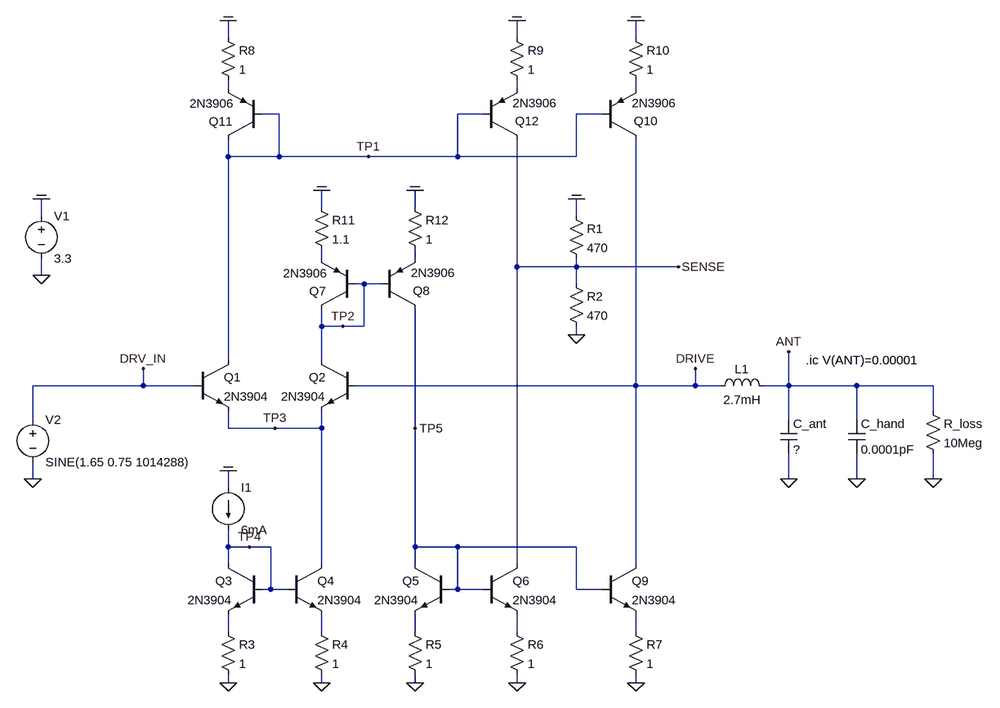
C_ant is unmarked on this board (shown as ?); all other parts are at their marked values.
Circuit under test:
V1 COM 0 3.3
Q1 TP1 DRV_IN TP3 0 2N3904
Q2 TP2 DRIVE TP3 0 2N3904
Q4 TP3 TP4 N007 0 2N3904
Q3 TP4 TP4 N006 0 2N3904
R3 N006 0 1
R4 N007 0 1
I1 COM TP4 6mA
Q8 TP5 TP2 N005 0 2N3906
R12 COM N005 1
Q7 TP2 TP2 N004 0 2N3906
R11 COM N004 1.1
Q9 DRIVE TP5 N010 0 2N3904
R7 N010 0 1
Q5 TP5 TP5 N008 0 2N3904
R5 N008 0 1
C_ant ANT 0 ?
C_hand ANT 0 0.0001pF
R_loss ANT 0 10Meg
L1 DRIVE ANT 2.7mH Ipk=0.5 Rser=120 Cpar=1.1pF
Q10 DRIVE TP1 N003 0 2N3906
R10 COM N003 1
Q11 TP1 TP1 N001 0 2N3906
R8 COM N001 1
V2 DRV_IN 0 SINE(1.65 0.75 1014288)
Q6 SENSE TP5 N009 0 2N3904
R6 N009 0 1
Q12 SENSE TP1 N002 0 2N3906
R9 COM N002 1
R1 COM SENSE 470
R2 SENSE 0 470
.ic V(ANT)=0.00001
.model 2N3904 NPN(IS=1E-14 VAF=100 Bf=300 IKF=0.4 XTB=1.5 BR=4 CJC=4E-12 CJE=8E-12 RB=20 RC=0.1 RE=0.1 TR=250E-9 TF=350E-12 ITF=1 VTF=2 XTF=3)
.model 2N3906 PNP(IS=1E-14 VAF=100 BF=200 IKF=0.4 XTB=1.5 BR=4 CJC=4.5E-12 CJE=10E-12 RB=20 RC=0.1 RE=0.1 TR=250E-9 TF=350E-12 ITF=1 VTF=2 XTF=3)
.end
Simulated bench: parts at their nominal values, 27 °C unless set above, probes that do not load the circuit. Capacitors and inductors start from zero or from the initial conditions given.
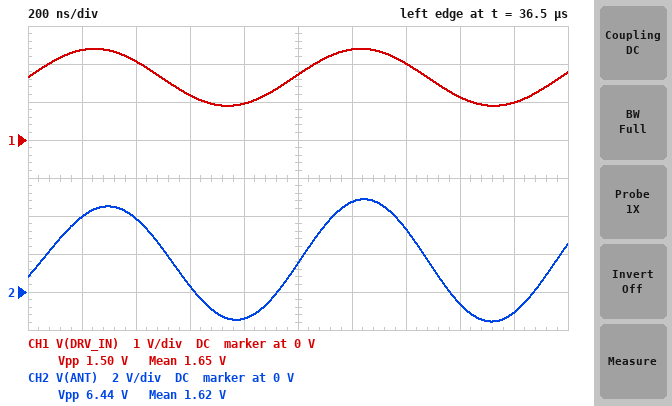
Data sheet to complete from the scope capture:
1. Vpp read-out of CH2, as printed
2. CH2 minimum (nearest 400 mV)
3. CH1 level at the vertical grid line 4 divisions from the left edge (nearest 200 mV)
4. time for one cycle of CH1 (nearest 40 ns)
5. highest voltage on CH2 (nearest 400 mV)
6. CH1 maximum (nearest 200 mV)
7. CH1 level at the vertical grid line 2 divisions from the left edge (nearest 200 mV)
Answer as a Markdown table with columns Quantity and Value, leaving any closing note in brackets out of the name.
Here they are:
| Quantity | Value |
|---|---|
| Vpp read-out of CH2, as printed | 6.44 V |
| CH2 minimum | -1.6 V |
| CH1 level at the vertical grid line 4 divisions from the left edge | 1.0 V |
| time for one cycle of CH1 | 1.00 µs |
| highest voltage on CH2 | 4.8 V |
| CH1 maximum | 2.4 V |
| CH1 level at the vertical grid line 2 divisions from the left edge | 2.0 V |
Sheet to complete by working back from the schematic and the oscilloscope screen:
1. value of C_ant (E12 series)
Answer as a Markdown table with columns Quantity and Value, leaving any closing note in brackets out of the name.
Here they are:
| Quantity | Value |
|---|---|
| value of C_ant | 5.6 pF |
